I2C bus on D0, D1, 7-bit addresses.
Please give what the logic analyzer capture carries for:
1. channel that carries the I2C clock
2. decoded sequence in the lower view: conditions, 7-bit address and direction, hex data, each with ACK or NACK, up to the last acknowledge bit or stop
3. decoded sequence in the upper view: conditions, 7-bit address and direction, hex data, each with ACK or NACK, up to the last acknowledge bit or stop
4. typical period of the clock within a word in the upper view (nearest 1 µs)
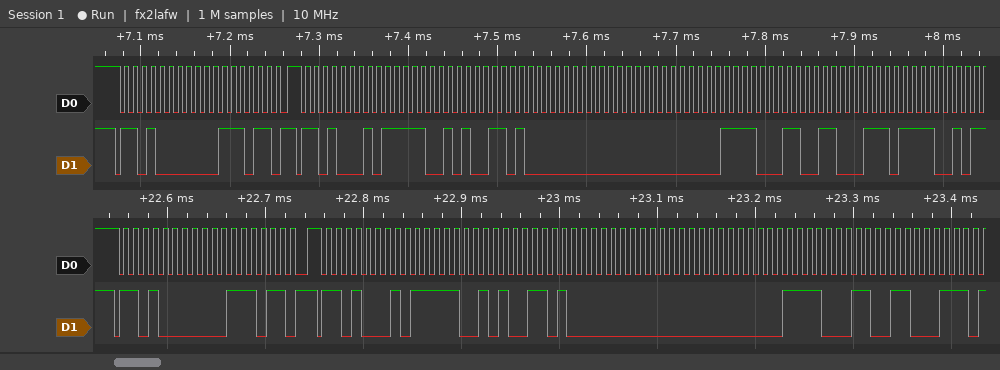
D0
start, address 68 write ACK, 3B ACK, repeated start, address 68 read ACK, F9 ACK, 9A ACK, 00 ACK, 00 ACK, 3C ACK, CC ACK
start, address 68 write ACK, 3B ACK, repeated start, address 68 read ACK, F9 ACK, 9A ACK, 00 ACK, 00 ACK, 3C ACK, CC ACK, EF ACK
10 µs
